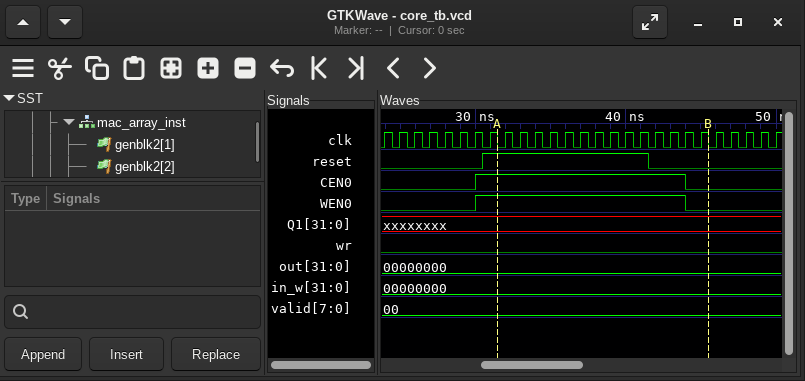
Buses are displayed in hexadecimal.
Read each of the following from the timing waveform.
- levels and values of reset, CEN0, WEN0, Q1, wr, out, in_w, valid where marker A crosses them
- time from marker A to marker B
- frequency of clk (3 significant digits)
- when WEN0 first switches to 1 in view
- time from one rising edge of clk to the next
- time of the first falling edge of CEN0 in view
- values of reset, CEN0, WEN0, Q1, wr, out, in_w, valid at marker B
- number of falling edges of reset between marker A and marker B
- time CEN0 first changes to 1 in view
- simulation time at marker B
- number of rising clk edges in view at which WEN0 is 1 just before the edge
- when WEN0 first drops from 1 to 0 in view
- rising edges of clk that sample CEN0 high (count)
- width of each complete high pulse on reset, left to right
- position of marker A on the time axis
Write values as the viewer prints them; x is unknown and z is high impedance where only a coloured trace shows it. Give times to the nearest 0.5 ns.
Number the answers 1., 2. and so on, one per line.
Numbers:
1. reset=1, CEN0=1, WEN0=1, Q1=xxxxxxxx, wr=0, out=00000000, in_w=00000000, valid=00
2. 14 ns
3. 1.00 GHz
4. 30 ns
5. 1 ns
6. 44 ns
7. reset=0, CEN0=0, WEN0=0, Q1=xxxxxxxx, wr=0, out=00000000, in_w=00000000, valid=00
8. 1
9. 30 ns
10. 45.5 ns
11. 14
12. 44 ns
13. 14
14. 11 ns
15. 31.5 ns
